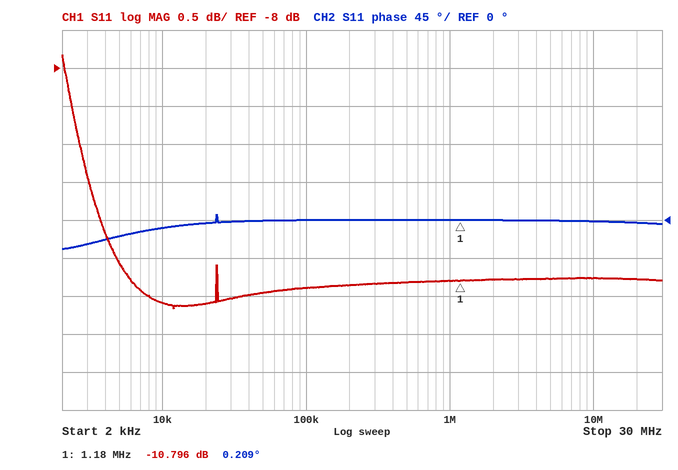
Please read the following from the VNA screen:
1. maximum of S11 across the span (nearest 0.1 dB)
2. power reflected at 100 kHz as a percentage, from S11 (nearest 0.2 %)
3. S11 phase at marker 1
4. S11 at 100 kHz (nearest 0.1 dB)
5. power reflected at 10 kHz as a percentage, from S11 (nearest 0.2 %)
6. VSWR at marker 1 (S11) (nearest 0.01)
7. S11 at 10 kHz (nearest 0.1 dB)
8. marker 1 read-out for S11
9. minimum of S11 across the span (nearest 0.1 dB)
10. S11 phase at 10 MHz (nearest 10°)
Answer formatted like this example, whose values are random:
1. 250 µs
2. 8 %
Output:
1. -7.8 dB
2. 8.2 %
3. 0.209°
4. -10.9 dB
5. 7.8 %
6. 1.81
7. -11.1 dB
8. -10.796 dB
9. -11.2 dB
10. 0°
